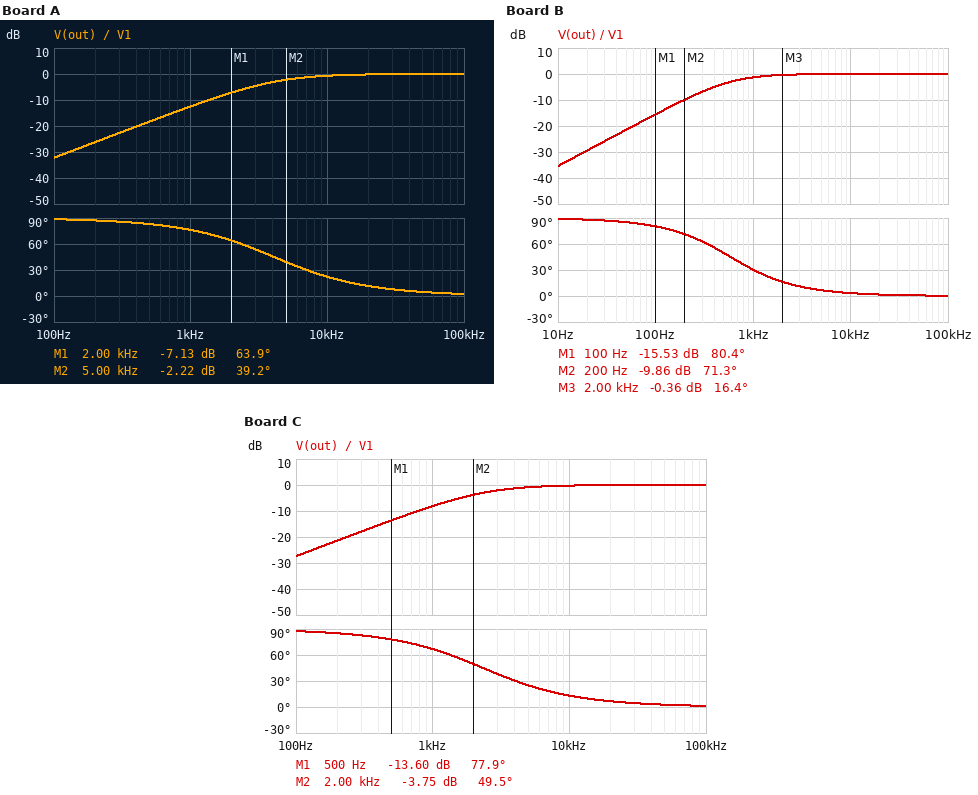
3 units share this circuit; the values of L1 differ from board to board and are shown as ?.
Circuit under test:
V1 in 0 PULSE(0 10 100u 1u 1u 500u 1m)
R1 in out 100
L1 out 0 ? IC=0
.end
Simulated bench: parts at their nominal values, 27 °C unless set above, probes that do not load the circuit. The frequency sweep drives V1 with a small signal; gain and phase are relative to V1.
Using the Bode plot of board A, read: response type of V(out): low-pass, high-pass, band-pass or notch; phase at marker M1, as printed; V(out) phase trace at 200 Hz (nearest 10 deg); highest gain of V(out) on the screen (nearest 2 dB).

high-pass
63.9 deg
90 deg
0 dB
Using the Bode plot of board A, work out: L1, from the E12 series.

3.9 mH
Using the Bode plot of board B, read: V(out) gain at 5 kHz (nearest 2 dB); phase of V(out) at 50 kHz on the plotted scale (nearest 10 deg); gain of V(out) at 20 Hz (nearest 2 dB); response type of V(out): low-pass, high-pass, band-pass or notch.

0 dB
0 deg
-30 dB
high-pass
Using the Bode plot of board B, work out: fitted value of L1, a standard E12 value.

27 mH
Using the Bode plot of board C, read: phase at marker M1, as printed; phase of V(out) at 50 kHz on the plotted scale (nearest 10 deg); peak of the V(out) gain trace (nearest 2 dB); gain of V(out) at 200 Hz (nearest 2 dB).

77.9 deg
0 deg
0 dB
-22 dB
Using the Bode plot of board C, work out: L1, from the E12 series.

6.8 mH
